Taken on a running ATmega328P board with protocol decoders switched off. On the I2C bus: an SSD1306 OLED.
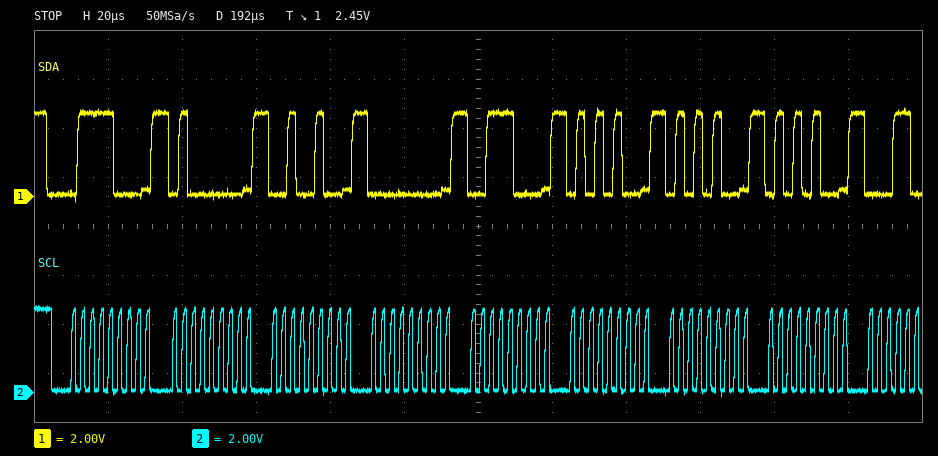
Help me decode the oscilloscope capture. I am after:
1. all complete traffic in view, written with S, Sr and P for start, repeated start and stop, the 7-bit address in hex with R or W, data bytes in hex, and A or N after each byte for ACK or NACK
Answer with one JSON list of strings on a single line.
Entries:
["S 3CW A 40 A 24 A 00 A 38 A 54 A 54 A 54 A"]
